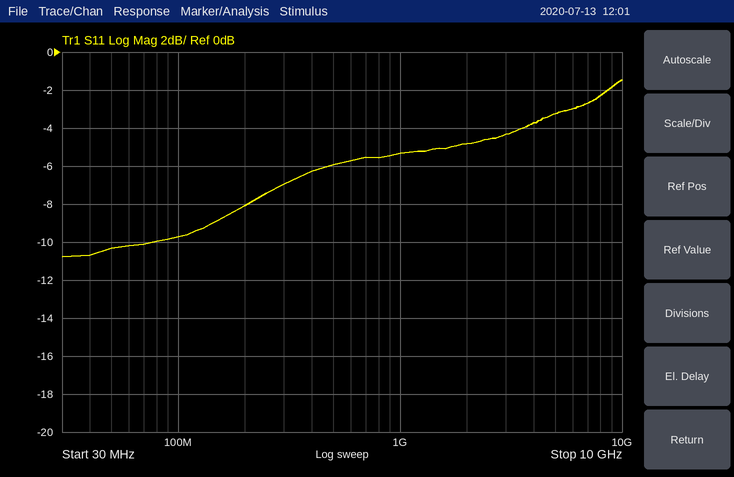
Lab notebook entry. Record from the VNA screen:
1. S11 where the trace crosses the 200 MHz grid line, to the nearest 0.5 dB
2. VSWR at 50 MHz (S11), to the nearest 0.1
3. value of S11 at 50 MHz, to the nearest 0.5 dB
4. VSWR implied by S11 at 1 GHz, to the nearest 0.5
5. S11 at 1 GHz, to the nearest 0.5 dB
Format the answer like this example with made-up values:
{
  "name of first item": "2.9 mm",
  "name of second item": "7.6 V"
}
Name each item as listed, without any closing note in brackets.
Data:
{
  "S11 where the trace crosses the 200 MHz grid line, to the nearest 0.5 dB": "-8.0 dB",
  "VSWR at 50 MHz (S11), to the nearest 0.1": "1.9",
  "value of S11 at 50 MHz, to the nearest 0.5 dB": "-10.5 dB",
  "VSWR implied by S11 at 1 GHz, to the nearest 0.5": "3.5",
  "S11 at 1 GHz, to the nearest 0.5 dB": "-5.5 dB"
}
